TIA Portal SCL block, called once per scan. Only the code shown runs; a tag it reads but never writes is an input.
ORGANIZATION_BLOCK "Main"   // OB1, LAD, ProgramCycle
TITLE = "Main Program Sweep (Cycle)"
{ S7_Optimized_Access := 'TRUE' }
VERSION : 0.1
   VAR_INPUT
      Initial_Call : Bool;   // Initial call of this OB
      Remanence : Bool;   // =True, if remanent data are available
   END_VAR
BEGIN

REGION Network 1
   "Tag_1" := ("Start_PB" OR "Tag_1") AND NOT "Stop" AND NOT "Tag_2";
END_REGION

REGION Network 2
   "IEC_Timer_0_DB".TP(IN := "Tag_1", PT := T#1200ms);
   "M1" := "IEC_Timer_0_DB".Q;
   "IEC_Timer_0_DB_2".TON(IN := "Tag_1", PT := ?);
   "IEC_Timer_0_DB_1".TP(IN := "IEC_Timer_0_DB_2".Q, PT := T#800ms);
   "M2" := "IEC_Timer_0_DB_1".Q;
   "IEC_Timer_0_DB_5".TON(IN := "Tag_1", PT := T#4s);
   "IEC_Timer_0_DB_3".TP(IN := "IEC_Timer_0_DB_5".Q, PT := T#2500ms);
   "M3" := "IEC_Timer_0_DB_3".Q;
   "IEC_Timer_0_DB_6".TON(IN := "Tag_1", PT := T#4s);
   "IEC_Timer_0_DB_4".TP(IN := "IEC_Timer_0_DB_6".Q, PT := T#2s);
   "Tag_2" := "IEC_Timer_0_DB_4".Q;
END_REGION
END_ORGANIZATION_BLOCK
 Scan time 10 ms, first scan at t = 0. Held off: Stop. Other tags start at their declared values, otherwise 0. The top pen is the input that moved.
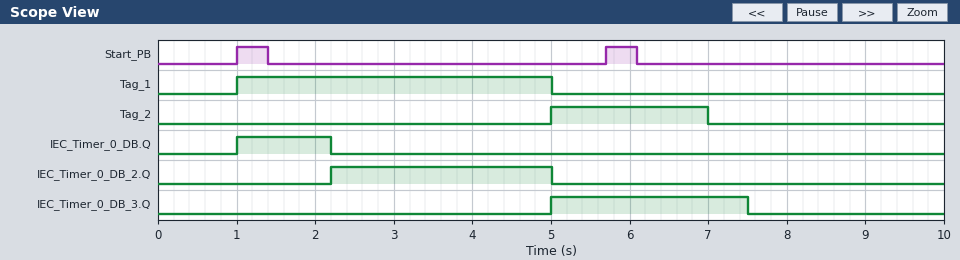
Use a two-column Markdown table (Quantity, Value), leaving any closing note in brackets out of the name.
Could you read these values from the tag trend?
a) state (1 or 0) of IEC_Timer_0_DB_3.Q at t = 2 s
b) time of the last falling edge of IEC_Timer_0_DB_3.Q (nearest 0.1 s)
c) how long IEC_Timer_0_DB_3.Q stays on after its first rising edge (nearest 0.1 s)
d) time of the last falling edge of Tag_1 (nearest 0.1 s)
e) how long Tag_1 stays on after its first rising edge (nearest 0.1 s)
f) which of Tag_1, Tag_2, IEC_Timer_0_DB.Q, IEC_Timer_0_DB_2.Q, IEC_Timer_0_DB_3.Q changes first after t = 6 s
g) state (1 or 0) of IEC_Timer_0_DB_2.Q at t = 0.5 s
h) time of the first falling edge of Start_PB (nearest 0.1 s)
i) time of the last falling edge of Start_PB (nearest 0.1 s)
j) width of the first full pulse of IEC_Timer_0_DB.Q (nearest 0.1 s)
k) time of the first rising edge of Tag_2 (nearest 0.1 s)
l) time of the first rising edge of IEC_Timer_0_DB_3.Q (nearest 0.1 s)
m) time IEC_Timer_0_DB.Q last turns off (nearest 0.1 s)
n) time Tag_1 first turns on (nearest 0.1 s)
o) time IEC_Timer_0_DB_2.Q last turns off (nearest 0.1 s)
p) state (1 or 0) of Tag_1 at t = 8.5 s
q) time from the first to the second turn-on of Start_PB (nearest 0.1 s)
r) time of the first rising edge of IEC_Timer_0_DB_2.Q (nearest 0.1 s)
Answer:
| Quantity | Value |
|---|---|
| state (1 or 0) of IEC_Timer_0_DB_3.Q at t = 2 s | 0 |
| time of the last falling edge of IEC_Timer_0_DB_3.Q | 7.5 s |
| how long IEC_Timer_0_DB_3.Q stays on after its first rising edge | 2.5 s |
| time of the last falling edge of Tag_1 | 5.0 s |
| how long Tag_1 stays on after its first rising edge | 4.0 s |
| which of Tag_1, Tag_2, IEC_Timer_0_DB.Q, IEC_Timer_0_DB_2.Q, IEC_Timer_0_DB_3.Q changes first after t = 6 s | Tag_2 |
| state (1 or 0) of IEC_Timer_0_DB_2.Q at t = 0.5 s | 0 |
| time of the first falling edge of Start_PB | 1.4 s |
| time of the last falling edge of Start_PB | 6.1 s |
| width of the first full pulse of IEC_Timer_0_DB.Q | 1.2 s |
| time of the first rising edge of Tag_2 | 5.0 s |
| time of the first rising edge of IEC_Timer_0_DB_3.Q | 5.0 s |
| time IEC_Timer_0_DB.Q last turns off | 2.2 s |
| time Tag_1 first turns on | 1.0 s |
| time IEC_Timer_0_DB_2.Q last turns off | 5.0 s |
| state (1 or 0) of Tag_1 at t = 8.5 s | 0 |
| time from the first to the second turn-on of Start_PB | 4.7 s |
| time of the first rising edge of IEC_Timer_0_DB_2.Q | 2.2 s |
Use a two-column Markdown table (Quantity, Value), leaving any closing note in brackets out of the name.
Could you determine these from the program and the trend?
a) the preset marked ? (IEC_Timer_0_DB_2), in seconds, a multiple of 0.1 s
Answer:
| Quantity | Value |
|---|---|
| the preset marked ? (IEC_Timer_0_DB_2), in seconds, a multiple of 0.1 s | 1.2 s |
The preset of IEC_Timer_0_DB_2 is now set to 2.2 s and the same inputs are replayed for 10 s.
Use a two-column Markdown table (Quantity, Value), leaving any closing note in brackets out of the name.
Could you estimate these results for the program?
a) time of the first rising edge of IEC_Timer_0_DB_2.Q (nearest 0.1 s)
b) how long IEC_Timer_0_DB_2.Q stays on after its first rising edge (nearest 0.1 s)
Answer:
| Quantity | Value |
|---|---|
| time of the first rising edge of IEC_Timer_0_DB_2.Q | 3.2 s |
| how long IEC_Timer_0_DB_2.Q stays on after its first rising edge | 1.8 s |
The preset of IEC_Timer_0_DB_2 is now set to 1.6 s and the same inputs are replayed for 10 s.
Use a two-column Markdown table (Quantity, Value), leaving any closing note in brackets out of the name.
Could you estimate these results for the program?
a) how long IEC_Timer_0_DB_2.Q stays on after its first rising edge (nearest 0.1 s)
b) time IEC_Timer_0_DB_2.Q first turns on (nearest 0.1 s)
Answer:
| Quantity | Value |
|---|---|
| how long IEC_Timer_0_DB_2.Q stays on after its first rising edge | 2.4 s |
| time IEC_Timer_0_DB_2.Q first turns on | 2.6 s |
